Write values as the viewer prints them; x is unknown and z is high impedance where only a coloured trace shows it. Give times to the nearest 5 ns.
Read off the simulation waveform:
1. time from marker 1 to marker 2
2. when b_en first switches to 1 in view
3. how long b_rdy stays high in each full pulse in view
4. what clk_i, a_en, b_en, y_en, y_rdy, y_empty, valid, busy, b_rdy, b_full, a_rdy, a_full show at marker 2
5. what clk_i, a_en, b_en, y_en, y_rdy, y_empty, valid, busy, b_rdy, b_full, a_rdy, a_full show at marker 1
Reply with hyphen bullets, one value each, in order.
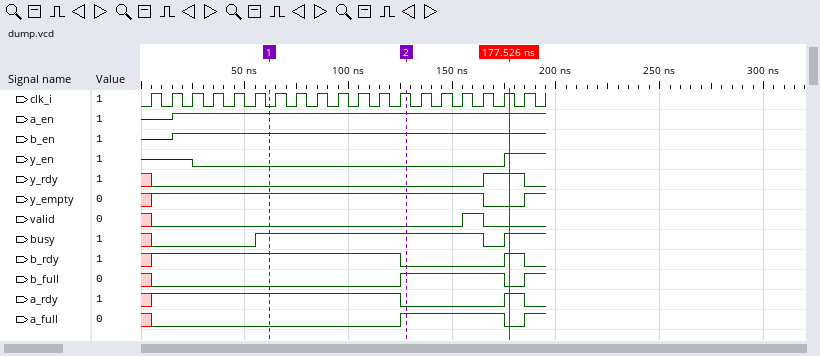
- 65 ns
- 15 ns
- 10 ns
- clk_i=1, a_en=1, b_en=1, y_en=0, y_rdy=0, y_empty=1, valid=0, busy=1, b_rdy=0, b_full=1, a_rdy=0, a_full=1
- clk_i=0, a_en=1, b_en=1, y_en=0, y_rdy=0, y_empty=1, valid=0, busy=1, b_rdy=1, b_full=0, a_rdy=1, a_full=0
